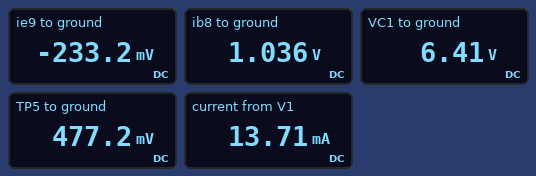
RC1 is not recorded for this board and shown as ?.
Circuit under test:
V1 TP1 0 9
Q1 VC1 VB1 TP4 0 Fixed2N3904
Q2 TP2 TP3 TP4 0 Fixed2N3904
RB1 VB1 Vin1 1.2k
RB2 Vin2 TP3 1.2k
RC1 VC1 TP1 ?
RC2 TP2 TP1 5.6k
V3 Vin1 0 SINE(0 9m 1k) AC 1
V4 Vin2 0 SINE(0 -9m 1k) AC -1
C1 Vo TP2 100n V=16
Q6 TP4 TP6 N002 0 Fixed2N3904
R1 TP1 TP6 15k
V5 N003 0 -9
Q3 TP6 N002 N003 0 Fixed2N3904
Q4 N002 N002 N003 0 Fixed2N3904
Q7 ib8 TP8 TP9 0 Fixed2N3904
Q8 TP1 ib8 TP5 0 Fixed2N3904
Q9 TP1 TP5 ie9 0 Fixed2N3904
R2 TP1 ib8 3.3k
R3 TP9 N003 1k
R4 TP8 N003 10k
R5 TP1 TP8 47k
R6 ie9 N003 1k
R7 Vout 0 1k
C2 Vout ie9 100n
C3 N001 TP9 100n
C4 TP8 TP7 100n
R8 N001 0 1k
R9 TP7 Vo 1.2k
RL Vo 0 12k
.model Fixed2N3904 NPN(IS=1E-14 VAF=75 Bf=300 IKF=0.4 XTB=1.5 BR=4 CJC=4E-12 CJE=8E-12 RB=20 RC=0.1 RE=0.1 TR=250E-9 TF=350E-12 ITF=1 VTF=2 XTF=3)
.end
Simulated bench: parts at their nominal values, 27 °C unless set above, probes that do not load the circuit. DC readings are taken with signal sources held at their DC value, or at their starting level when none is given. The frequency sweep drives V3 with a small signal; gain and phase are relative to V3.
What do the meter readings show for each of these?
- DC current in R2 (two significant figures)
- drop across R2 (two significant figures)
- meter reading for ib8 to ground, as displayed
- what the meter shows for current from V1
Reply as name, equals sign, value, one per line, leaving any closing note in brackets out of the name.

DC current in R2 = 2.4 mA
drop across R2 = 8.0 V
meter reading for ib8 to ground, as displayed = 1.036 V
what the meter shows for current from V1 = 13.71 mA
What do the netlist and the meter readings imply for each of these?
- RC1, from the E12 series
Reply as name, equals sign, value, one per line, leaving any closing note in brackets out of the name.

RC1, from the E12 series = 4.7 kΩ
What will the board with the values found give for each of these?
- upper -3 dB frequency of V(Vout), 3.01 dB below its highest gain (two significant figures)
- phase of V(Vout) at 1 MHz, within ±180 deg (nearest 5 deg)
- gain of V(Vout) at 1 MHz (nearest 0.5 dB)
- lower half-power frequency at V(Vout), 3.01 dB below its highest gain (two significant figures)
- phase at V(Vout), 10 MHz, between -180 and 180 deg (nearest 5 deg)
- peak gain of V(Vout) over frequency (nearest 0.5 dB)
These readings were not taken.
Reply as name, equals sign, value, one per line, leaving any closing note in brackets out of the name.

upper -3 dB frequency of V(Vout), 3.01 dB below its highest gain = 740 kHz
phase of V(Vout) at 1 MHz, within ±180 deg = 110 deg
gain of V(Vout) at 1 MHz = 44.5 dB
lower half-power frequency at V(Vout), 3.01 dB below its highest gain = 2.2 kHz
phase at V(Vout), 10 MHz, between -180 and 180 deg = 15 deg
peak gain of V(Vout) over frequency = 49.0 dB
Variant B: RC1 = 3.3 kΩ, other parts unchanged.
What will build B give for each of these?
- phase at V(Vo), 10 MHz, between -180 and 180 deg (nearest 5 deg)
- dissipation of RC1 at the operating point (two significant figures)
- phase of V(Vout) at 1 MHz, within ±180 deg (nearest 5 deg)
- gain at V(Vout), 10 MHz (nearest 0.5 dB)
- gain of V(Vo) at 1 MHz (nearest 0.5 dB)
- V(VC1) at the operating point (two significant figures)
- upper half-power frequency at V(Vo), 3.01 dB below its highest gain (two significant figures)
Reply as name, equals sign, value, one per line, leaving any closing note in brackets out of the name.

phase at V(Vo), 10 MHz, between -180 and 180 deg = -90 deg
dissipation of RC1 at the operating point = 1.0 mW
phase of V(Vout) at 1 MHz, within ±180 deg = 115 deg
gain at V(Vout), 10 MHz = 18.5 dB
gain of V(Vo) at 1 MHz = 30.5 dB
V(VC1) at the operating point = 7.2 V
upper half-power frequency at V(Vo), 3.01 dB below its highest gain = 870 kHz
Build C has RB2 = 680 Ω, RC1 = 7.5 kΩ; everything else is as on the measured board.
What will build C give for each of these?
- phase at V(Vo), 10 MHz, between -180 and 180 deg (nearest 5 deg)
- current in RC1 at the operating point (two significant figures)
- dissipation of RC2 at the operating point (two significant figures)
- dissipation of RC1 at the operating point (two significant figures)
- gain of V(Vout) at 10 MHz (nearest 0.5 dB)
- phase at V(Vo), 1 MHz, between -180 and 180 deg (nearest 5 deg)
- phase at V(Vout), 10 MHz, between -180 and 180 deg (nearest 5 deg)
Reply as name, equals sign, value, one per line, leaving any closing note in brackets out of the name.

phase at V(Vo), 10 MHz, between -180 and 180 deg = -70 deg
current in RC1 at the operating point = 540 µA
dissipation of RC2 at the operating point = 1.8 mW
dissipation of RC1 at the operating point = 2.2 mW
gain of V(Vout) at 10 MHz = 16.0 dB
phase at V(Vo), 1 MHz, between -180 and 180 deg = -65 deg
phase at V(Vout), 10 MHz, between -180 and 180 deg = 30 deg
